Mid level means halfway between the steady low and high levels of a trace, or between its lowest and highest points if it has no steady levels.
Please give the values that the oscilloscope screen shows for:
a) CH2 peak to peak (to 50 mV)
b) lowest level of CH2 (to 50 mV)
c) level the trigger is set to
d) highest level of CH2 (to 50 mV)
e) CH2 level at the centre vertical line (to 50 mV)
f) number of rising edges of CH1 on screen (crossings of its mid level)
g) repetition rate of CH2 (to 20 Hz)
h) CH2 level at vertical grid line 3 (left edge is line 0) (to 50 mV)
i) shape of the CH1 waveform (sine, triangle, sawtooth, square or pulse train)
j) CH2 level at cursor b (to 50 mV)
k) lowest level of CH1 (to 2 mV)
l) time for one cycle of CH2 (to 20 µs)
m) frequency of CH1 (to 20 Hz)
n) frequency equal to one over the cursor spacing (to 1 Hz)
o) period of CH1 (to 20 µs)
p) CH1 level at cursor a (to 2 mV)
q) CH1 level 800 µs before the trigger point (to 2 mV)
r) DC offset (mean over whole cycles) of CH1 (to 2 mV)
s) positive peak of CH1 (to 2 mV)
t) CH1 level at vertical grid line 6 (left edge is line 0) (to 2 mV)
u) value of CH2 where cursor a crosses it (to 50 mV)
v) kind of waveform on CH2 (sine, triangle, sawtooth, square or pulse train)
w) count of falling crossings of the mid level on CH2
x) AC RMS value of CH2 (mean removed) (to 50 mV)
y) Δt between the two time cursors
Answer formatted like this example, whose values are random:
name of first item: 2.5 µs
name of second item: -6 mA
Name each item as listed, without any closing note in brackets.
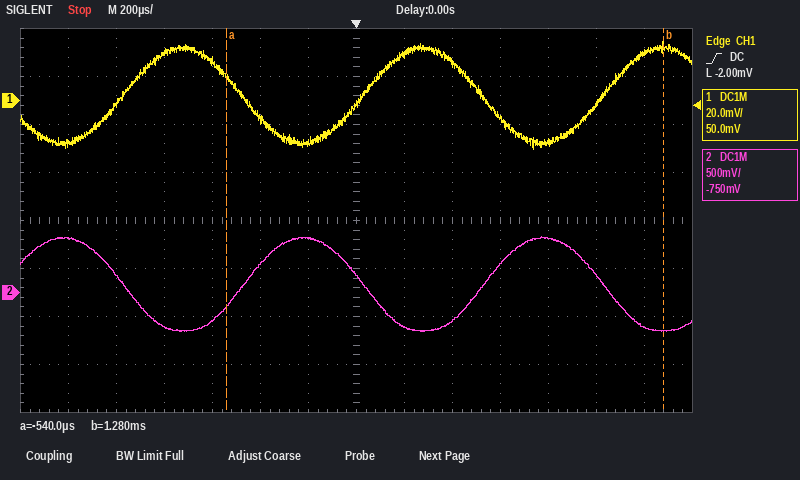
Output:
CH2 peak to peak: 1.00 V
lowest level of CH2: -400 mV
level the trigger is set to: -2.00 mV
highest level of CH2: 600 mV
CH2 level at the centre vertical line: 200 mV
number of rising edges of CH1 on screen: 3
repetition rate of CH2: 1.00 kHz
CH2 level at vertical grid line 3 (left edge is line 0): -350 mV
shape of the CH1 waveform: sine
CH2 level at cursor b: -400 mV
lowest level of CH1: -20 mV
time for one cycle of CH2: 1.00 ms
frequency of CH1: 1.00 kHz
frequency equal to one over the cursor spacing: 549 Hz
period of CH1: 1.00 ms
CH1 level at cursor a: 10 mV
CH1 level 800 µs before the trigger point: 20 mV
DC offset (mean over whole cycles) of CH1: 2 mV
positive peak of CH1: 24 mV
CH1 level at vertical grid line 6 (left edge is line 0): -18 mV
value of CH2 where cursor a crosses it: -150 mV
kind of waveform on CH2: sine
count of falling crossings of the mid level on CH2: 3
AC RMS value of CH2 (mean removed): 350 mV
Δt between the two time cursors: 1.82 ms
